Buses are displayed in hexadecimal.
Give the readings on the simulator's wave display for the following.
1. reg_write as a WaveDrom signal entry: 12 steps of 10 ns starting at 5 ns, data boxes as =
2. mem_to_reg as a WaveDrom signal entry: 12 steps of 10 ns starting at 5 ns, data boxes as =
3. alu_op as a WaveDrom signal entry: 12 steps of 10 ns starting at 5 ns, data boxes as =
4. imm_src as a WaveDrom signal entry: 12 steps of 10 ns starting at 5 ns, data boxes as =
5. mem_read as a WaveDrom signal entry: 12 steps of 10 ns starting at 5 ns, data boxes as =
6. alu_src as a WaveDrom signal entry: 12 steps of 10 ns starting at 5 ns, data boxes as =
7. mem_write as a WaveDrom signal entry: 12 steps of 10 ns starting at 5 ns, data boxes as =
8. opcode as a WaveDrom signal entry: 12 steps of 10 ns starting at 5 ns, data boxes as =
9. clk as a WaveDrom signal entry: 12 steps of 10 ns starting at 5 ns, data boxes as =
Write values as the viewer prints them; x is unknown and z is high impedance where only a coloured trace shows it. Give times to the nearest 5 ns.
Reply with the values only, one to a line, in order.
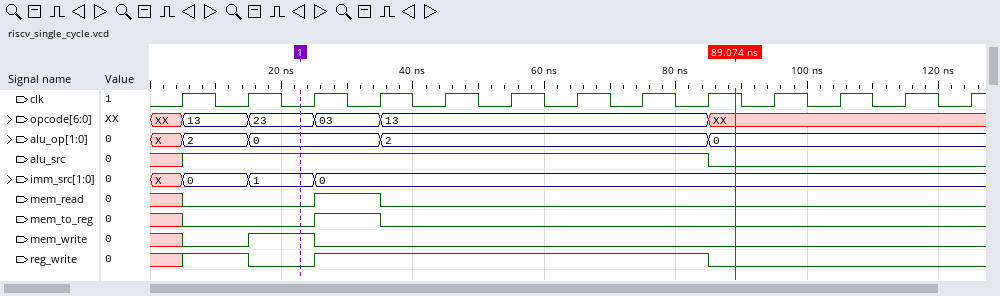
{name: 'reg_write', wave: '101.....0...'}
{name: 'mem_to_reg', wave: '0.10........'}
{name: 'alu_op', wave: '==.=....=...', data: '2 0 2 0'}
{name: 'imm_src', wave: '===.........', data: '0 1 0'}
{name: 'mem_read', wave: '0.10........'}
{name: 'alu_src', wave: '1.......0...'}
{name: 'mem_write', wave: '010.........'}
{name: 'opcode', wave: '====....x...', data: '13 23 03 13'}
{name: 'clk', wave: 'p...........'}
